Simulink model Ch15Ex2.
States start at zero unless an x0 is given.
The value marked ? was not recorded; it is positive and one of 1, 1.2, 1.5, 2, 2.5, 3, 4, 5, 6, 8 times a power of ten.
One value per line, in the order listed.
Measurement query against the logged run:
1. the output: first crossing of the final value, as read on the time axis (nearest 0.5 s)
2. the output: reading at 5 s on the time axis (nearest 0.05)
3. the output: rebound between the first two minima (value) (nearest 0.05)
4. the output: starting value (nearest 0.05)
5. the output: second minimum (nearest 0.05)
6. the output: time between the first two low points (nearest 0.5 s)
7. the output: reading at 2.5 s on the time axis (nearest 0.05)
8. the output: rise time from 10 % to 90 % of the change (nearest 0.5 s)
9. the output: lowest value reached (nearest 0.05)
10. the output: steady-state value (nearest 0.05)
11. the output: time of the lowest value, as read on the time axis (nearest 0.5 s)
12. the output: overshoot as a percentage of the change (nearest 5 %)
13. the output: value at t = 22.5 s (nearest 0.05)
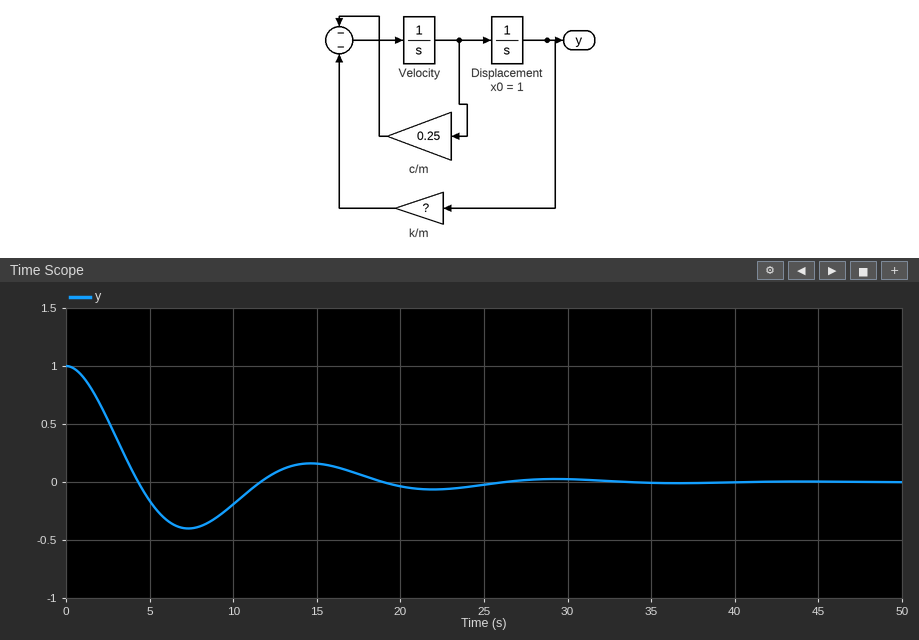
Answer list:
4.5 s
-0.15
0.15
1.00
-0.05
14.5 s
0.55
3.0 s
-0.40
0.00
7.5 s
40 %
-0.05
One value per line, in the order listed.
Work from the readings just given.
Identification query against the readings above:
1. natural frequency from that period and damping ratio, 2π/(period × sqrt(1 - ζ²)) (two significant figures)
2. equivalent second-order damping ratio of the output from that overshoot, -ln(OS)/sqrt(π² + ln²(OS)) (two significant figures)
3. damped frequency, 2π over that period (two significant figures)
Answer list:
0.45 rad/s
0.28
0.43 rad/s
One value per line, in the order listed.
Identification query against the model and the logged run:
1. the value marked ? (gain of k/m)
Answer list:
0.2
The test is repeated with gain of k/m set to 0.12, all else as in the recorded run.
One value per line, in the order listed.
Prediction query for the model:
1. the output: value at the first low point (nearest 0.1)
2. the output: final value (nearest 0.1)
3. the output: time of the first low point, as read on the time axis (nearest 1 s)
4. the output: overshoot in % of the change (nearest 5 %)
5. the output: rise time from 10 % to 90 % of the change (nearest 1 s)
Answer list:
-0.3
0.0
10 s
30 %
4 s
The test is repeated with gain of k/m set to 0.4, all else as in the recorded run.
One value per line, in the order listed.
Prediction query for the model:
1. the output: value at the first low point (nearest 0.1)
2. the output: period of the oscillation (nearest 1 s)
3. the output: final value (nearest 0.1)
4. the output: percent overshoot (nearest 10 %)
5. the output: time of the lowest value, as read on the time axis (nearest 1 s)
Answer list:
-0.5
10 s
0.0
50 %
5 s
